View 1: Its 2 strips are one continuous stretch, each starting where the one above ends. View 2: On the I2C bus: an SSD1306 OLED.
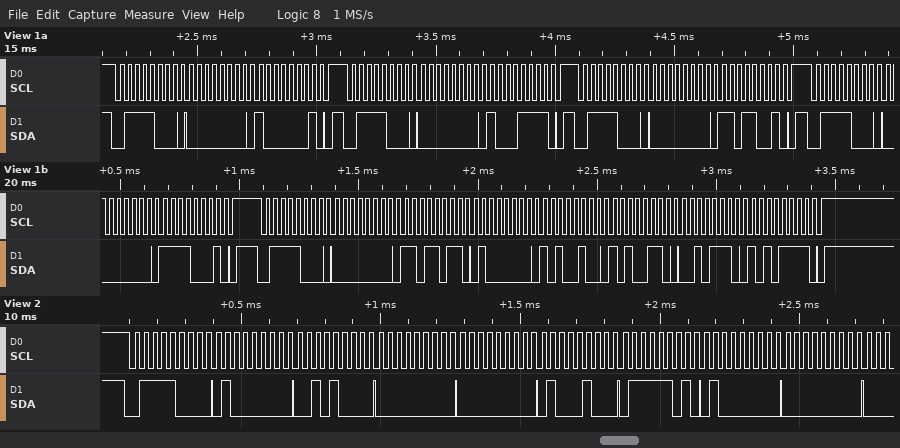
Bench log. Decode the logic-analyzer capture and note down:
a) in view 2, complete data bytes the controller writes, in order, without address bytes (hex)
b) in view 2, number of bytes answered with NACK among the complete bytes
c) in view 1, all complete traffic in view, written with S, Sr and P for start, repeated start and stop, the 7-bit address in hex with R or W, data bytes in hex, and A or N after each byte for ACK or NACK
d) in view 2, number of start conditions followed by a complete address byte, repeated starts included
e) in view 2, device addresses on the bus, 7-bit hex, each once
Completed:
40 28 00 00 44 7D 40 00
0
S 3CW A 00 A 81 A P S 3CW A 00 A 8F A P S 3CW A 00 A D9 A P S 3CW A 00 A F1 A P S 3CW A 00 A DB A 40 A A4 A A6 A 2E A AF A P
1
0x3C
